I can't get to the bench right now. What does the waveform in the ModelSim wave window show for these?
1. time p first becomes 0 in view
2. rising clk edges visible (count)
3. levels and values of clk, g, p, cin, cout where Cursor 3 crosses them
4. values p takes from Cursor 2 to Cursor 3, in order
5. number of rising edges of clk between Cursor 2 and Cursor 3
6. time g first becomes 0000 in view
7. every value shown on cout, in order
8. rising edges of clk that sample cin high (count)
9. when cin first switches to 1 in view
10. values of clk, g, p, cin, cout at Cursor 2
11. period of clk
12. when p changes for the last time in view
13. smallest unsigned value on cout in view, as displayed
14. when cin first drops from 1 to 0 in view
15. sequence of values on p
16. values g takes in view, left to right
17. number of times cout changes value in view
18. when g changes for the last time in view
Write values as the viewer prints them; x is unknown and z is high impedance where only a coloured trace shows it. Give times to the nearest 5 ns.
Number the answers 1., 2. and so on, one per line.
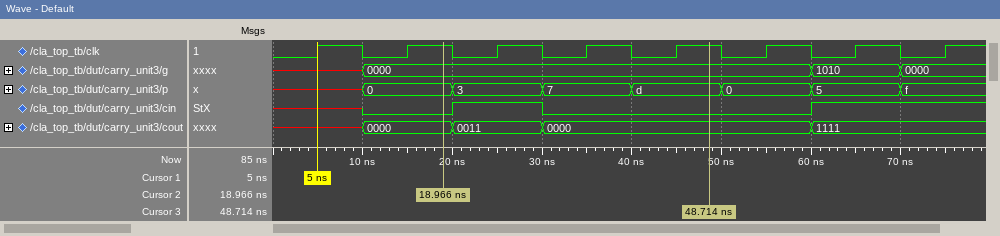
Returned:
1. 10 ns
2. 8
3. clk=1, g=0000, p=d, cin=0, cout=0000
4. 0, 3, 7, d
5. 3
6. 10 ns
7. x, 0000, 0011, 0000, 1111
8. 3
9. 20 ns
10. clk=1, g=0000, p=0, cin=0, cout=0000
11. 10 ns
12. 70 ns
13. 0000
14. 30 ns
15. x, 0, 3, 7, d, 0, 5, f
16. x, 0000, 1010, 0000
17. 4
18. 70 ns
